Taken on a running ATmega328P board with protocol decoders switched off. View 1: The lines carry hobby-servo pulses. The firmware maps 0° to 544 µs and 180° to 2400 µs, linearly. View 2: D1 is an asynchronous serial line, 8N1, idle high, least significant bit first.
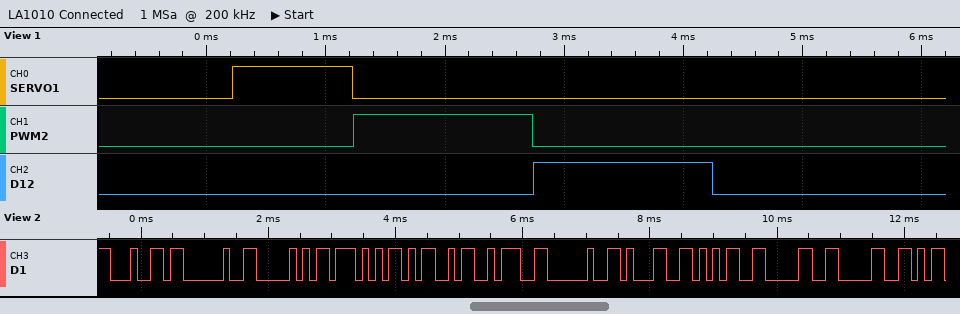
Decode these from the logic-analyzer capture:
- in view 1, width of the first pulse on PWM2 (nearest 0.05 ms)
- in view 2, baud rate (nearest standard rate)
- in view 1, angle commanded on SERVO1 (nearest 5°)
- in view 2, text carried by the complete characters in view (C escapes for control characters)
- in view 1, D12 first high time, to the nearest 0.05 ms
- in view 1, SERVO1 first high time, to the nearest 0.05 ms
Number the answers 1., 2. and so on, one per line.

1. 1.50 ms
2. 9600 baud
3. 45°
4. "d PWM: 1500"
5. 1.50 ms
6. 1.00 ms
